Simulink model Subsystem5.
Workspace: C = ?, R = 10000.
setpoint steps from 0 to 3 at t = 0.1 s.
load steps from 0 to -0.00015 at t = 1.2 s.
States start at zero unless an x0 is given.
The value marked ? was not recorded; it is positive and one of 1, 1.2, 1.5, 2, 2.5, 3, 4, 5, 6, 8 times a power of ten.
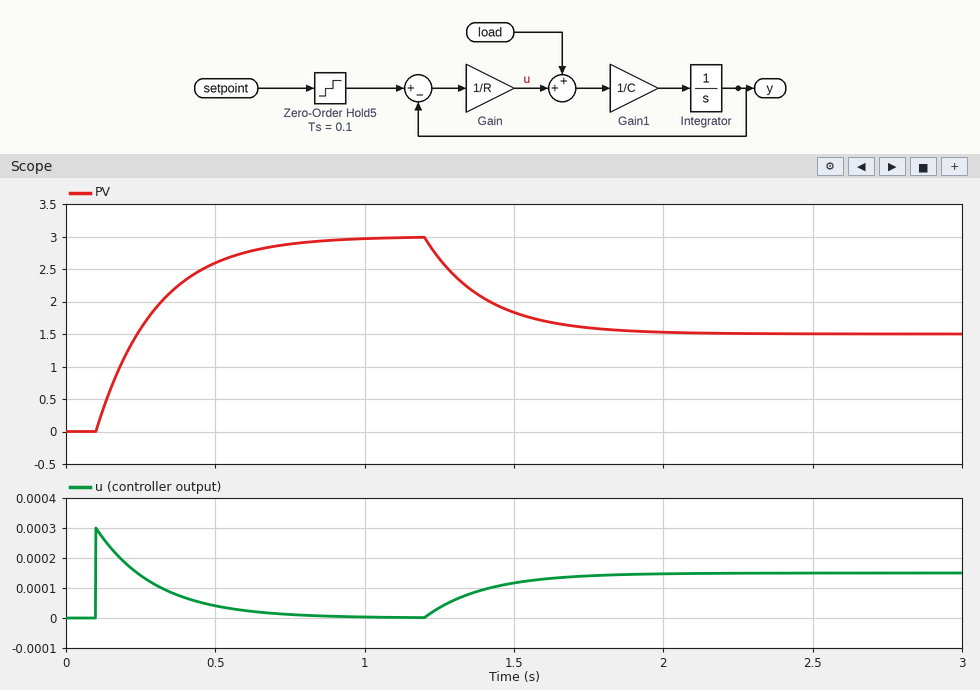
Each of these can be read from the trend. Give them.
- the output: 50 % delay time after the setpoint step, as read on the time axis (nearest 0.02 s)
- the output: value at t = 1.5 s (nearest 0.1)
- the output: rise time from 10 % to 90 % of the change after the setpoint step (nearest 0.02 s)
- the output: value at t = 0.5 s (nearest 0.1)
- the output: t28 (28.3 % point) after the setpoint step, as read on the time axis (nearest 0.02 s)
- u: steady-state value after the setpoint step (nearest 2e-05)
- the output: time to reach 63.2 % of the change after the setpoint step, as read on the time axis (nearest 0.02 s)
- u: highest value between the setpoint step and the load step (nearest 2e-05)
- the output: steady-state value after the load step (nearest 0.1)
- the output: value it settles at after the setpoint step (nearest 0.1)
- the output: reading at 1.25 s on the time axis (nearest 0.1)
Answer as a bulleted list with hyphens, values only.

- 0.24 s
- 1.8
- 0.44 s
- 2.6
- 0.16 s
- 0.00000
- 0.30 s
- 0.00030
- 1.5
- 3.0
- 2.7
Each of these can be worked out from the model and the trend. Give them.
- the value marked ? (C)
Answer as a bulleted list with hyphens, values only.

- 2e-05
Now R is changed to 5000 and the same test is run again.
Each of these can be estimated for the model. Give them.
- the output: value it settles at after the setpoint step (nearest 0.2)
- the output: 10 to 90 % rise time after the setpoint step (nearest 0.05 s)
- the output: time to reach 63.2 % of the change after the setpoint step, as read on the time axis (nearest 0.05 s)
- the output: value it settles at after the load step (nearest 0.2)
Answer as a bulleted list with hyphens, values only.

- 3.0
- 0.20 s
- 0.20 s
- 2.2
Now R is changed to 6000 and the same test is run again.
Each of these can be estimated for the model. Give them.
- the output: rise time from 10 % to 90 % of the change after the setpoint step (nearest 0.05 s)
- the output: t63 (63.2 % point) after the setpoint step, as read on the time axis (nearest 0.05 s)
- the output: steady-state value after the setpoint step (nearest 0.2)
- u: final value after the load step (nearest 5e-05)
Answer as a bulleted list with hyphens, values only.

- 0.25 s
- 0.20 s
- 3.0
- 0.00015
